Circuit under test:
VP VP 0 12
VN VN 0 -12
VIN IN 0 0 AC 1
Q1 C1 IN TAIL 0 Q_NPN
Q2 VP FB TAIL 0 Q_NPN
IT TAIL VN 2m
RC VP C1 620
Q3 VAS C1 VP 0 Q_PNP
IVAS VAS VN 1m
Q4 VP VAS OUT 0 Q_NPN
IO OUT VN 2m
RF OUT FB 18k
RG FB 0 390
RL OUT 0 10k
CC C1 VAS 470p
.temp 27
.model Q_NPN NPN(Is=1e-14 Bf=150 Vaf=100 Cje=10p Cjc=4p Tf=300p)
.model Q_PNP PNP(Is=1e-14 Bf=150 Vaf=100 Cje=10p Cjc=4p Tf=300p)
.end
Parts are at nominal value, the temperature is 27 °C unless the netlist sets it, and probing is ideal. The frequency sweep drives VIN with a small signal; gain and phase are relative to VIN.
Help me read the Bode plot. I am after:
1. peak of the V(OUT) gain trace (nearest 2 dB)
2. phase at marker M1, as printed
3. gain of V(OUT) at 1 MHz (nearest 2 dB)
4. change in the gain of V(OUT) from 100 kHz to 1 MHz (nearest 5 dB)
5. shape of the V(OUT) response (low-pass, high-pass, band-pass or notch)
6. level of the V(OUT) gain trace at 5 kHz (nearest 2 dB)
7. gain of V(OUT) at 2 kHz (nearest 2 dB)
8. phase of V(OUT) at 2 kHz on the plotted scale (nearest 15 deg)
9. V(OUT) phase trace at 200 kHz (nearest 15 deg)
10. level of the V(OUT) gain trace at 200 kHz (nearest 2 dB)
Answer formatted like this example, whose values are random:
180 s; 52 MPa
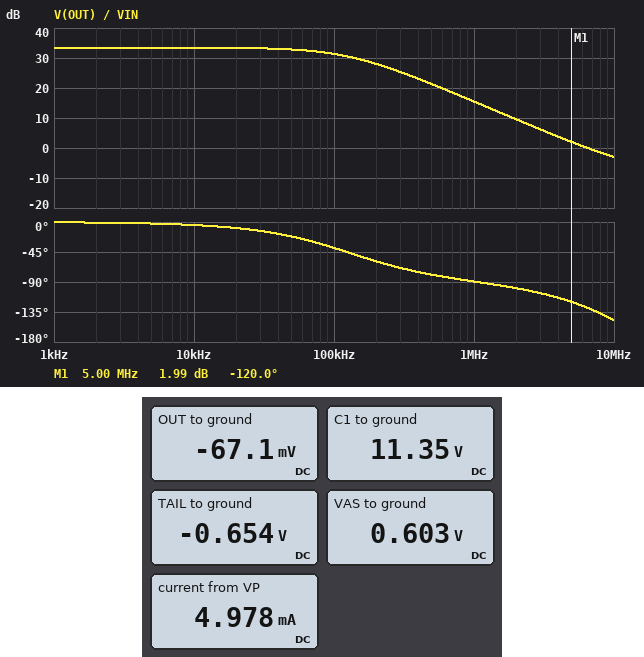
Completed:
34 dB; -120.0 deg; 16 dB; -15 dB; low-pass; 34 dB; 34 dB; 0 deg; -60 deg; 28 dB
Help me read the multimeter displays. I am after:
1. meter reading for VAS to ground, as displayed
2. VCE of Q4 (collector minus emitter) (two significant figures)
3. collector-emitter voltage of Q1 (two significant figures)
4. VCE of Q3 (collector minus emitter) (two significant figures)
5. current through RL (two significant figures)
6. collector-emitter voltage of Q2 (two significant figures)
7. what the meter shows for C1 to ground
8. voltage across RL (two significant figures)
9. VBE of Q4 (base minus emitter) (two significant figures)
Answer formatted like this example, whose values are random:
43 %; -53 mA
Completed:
0.603 V; 12 V; 12 V; -11 V; 6.7 µA; 13 V; 11.35 V; 67 mV; 670 mV
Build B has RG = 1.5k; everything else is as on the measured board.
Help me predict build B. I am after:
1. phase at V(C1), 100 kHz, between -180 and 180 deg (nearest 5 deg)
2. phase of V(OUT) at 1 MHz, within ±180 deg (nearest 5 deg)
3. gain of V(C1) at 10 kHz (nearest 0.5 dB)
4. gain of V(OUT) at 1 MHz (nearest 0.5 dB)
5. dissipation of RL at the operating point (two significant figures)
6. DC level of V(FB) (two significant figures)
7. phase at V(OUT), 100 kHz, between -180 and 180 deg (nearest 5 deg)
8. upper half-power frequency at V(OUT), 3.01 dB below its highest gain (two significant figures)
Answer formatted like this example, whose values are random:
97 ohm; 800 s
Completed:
-105 deg; -75 deg; -39.5 dB; 14.5 dB; 290 nW; -3.5 mV; -15 deg; 450 kHz
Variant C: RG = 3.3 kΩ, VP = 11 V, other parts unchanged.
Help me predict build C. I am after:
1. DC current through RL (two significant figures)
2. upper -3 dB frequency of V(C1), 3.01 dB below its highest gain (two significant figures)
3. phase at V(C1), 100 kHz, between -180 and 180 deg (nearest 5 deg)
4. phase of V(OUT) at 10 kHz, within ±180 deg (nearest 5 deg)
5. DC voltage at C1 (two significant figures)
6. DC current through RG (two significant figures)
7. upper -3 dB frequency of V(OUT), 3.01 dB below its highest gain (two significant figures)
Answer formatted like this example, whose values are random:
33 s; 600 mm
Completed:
7.7 µA; 5.3 MHz; -100 deg; 0 deg; 10 V; 1.1 µA; 920 kHz
